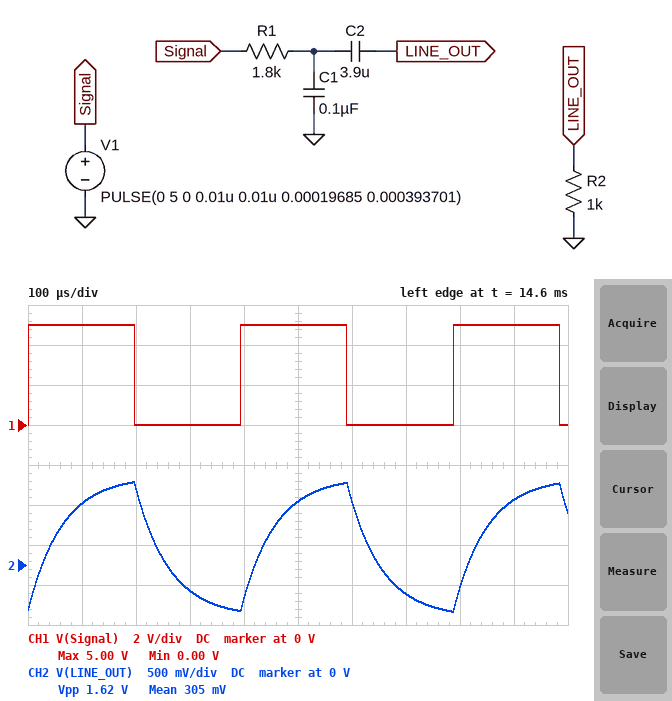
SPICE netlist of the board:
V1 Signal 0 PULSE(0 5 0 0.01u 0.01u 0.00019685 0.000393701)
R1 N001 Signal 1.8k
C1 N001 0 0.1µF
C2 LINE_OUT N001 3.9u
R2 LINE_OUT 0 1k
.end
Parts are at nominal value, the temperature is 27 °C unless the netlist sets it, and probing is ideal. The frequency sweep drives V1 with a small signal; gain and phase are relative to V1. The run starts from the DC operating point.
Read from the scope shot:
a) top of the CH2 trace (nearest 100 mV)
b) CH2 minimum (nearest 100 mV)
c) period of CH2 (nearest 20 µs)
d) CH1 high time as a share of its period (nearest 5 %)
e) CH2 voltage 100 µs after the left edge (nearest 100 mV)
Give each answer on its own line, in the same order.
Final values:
1.0 V
-600 mV
400 µs
50 %
800 mV
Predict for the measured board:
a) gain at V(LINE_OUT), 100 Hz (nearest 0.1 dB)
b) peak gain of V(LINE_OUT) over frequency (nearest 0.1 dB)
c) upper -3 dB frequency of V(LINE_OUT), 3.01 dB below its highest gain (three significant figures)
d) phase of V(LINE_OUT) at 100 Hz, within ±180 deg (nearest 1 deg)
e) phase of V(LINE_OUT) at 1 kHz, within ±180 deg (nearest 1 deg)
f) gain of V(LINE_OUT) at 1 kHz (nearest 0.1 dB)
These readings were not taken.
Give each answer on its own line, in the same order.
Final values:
-9.1 dB
-9.1 dB
2.53 kHz
6 deg
-21 deg
-9.7 dB
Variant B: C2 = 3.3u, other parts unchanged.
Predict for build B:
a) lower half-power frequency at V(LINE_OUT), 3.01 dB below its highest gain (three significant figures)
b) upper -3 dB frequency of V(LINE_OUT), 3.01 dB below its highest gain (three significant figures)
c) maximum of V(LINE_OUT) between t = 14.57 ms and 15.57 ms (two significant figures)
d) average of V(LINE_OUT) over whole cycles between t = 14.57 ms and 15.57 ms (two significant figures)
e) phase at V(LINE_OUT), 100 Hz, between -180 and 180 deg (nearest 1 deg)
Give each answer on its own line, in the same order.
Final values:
16.8 Hz
2.54 kHz
980 mV
180 mV
7 deg
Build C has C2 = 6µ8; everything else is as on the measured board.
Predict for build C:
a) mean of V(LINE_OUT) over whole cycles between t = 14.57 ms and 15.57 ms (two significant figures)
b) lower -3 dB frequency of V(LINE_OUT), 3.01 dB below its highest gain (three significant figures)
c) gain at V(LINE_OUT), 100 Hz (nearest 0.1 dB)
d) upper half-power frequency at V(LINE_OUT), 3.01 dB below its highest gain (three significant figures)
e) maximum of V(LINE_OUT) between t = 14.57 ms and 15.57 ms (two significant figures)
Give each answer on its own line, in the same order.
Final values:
400 mV
8.25 Hz
-9.0 dB
2.51 kHz
1.2 V
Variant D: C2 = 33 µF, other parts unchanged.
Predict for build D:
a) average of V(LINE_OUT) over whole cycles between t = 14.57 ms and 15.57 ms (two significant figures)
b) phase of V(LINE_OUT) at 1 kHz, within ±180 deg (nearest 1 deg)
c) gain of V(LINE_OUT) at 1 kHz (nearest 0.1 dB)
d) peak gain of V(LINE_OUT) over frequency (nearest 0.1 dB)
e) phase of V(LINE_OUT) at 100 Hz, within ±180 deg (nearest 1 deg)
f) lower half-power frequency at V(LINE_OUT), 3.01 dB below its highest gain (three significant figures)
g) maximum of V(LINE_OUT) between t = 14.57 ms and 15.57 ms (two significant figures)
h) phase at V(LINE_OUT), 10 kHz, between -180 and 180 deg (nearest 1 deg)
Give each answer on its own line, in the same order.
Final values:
760 mV
-22 deg
-9.6 dB
-9.0 dB
-1 deg
1.72 Hz
1.6 V
-76 deg
